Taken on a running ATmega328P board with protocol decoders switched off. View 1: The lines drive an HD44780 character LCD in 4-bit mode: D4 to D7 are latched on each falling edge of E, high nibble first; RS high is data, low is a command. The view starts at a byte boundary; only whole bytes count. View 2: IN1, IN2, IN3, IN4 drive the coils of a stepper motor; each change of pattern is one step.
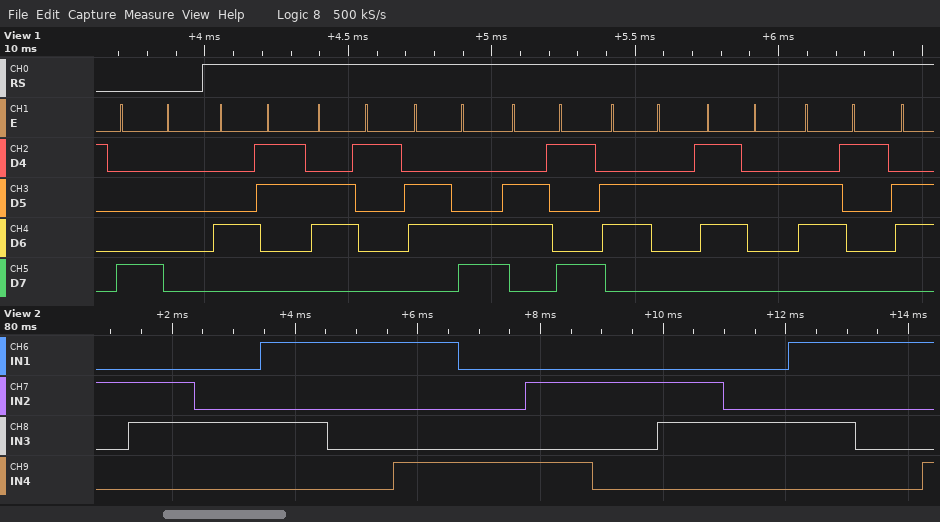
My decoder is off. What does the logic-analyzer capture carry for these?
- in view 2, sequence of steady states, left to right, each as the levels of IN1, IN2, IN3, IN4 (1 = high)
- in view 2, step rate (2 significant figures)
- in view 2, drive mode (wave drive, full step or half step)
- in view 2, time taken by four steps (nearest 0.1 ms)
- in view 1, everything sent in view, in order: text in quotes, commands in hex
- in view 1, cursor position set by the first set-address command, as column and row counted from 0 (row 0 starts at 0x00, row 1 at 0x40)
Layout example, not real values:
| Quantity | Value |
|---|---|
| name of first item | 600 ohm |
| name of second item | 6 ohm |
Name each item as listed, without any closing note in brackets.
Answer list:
| Quantity | Value |
|---|---|
| in view 2, sequence of steady states, left to right, each as the levels of IN1, IN2, IN3, IN4 | 0100 0110 0010 1010 1000 1001 0001 0101 0100 0110 0010 1010 1000 1001 |
| in view 2, step rate | 930 steps/s |
| in view 2, drive mode | half step |
| in view 2, time taken by four steps | 4.3 ms |
| in view 1, everything sent in view, in order: text in quotes, commands in hex | 0x80 "Calibra" |
| in view 1, cursor position set by the first set-address command, as column and row counted from 0 | column 0, row 0 |
